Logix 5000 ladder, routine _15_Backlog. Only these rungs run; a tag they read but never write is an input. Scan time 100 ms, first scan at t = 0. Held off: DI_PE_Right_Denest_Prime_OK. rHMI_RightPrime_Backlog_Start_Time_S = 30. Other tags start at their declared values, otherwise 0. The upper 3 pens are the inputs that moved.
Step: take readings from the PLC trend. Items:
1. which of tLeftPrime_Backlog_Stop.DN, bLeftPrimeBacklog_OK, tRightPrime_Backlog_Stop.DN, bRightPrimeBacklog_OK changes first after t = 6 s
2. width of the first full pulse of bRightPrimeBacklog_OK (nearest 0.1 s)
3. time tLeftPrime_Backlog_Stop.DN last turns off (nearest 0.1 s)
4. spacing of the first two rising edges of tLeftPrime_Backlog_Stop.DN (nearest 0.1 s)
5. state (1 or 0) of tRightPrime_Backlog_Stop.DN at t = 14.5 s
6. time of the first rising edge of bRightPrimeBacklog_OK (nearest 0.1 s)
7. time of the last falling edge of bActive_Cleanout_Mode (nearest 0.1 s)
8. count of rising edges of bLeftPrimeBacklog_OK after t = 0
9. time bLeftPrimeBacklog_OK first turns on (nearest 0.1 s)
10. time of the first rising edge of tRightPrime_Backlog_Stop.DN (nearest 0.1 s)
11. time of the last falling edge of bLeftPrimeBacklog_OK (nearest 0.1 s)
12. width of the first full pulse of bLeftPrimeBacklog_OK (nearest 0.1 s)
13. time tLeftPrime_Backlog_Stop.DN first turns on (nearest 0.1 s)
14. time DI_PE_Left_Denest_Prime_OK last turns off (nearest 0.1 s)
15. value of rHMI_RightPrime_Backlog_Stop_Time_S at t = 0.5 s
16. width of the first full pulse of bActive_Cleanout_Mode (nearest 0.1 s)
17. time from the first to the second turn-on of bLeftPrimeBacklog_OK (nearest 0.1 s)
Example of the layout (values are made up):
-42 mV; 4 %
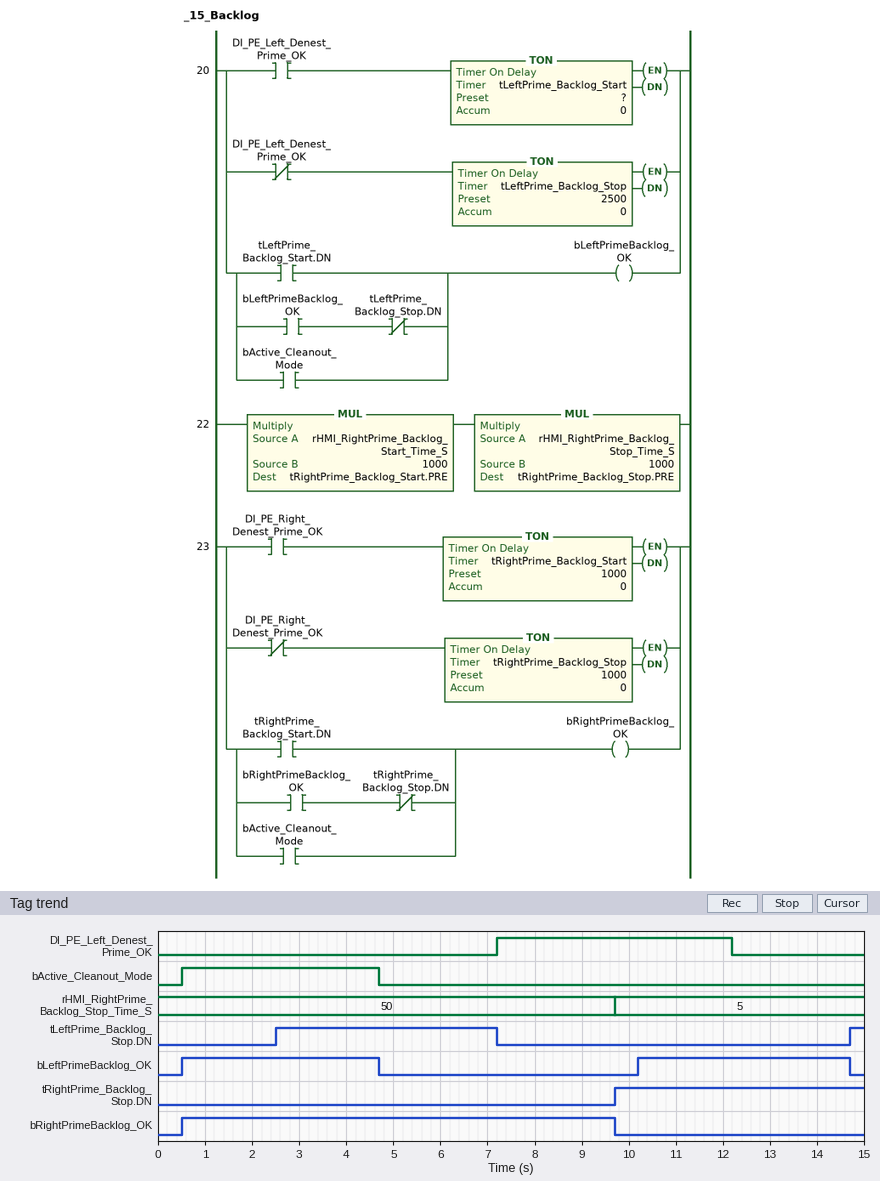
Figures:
tLeftPrime_Backlog_Stop.DN; 9.2 s; 7.2 s; 12.2 s; 1; 0.5 s; 4.7 s; 2; 0.5 s; 9.7 s; 14.7 s; 4.2 s; 2.5 s; 12.2 s; 50; 4.2 s; 9.7 s
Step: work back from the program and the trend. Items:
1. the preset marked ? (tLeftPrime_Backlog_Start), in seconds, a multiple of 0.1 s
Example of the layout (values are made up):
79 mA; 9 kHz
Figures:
3.0 s
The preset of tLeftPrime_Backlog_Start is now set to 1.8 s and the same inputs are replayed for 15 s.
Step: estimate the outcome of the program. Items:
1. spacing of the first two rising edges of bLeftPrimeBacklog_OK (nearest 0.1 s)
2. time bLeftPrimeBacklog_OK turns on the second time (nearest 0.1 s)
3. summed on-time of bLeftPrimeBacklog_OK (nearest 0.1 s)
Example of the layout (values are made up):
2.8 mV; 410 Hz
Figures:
8.5 s; 9.0 s; 9.9 s
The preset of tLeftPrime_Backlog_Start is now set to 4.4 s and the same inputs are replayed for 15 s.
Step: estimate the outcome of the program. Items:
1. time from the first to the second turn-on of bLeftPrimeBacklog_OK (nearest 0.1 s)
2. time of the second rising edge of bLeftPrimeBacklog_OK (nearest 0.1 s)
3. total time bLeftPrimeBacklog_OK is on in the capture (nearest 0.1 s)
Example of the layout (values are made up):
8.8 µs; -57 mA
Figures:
11.1 s; 11.6 s; 7.3 s
